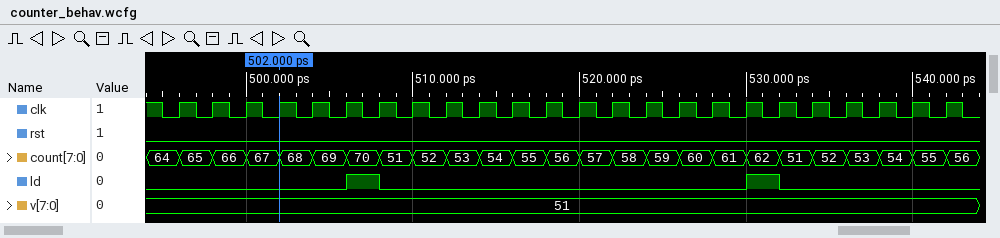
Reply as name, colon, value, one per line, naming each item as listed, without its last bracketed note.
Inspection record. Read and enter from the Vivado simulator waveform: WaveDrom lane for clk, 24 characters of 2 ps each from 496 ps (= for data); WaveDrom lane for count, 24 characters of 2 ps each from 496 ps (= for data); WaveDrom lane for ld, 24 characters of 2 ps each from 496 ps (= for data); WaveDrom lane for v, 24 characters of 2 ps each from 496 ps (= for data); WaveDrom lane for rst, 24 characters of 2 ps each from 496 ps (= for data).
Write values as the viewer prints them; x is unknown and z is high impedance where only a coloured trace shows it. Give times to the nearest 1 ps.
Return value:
WaveDrom lane for clk, 24 characters of 2 ps each from 496 ps: {name: 'clk', wave: 'p.......................'}
WaveDrom lane for count, 24 characters of 2 ps each from 496 ps: {name: 'count', wave: '========================', data: '65 66 67 68 69 70 51 52 53 54 55 56 57 58 59 60 61 62 51 52 53 54 55 56'}
WaveDrom lane for ld, 24 characters of 2 ps each from 496 ps: {name: 'ld', wave: '0....10..........10.....'}
WaveDrom lane for v, 24 characters of 2 ps each from 496 ps: {name: 'v', wave: '=.......................', data: '51'}
WaveDrom lane for rst, 24 characters of 2 ps each from 496 ps: {name: 'rst', wave: '0.......................'}
